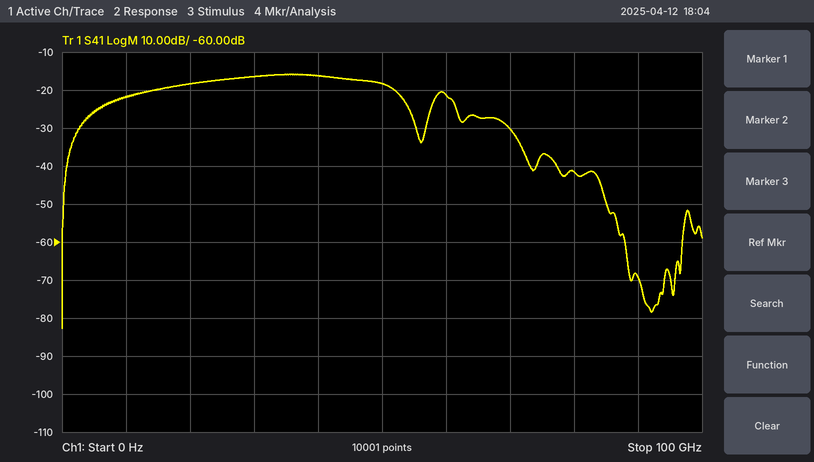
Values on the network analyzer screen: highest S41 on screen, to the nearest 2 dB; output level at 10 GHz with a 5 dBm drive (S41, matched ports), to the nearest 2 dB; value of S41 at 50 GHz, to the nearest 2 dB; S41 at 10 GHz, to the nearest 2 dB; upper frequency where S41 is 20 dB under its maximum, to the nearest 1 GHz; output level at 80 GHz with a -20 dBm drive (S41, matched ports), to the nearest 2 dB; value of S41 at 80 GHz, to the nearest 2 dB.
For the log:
-16 dB
-16 dBm
-18 dB
-22 dB
72 GHz
-62 dBm
-42 dB
